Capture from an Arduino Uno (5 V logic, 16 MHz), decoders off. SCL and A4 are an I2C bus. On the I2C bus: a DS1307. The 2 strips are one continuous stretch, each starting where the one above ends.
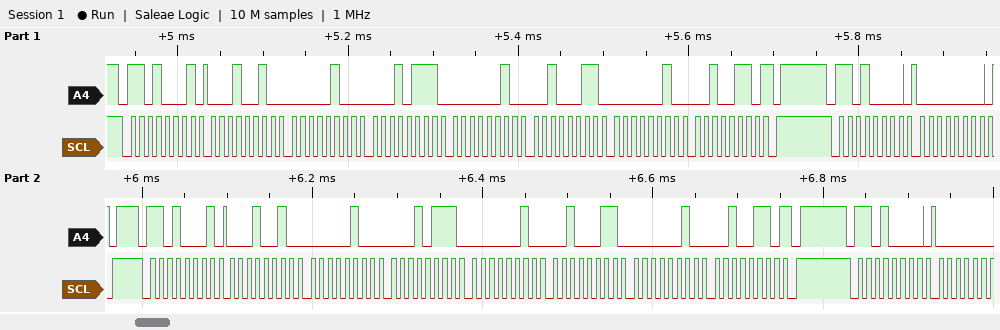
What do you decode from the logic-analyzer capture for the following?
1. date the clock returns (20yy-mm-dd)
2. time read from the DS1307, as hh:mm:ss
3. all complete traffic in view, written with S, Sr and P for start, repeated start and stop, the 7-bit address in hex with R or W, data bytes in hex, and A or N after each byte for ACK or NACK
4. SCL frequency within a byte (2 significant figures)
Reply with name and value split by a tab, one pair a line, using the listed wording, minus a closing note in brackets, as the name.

date the clock returns	2026-02-23
time read from the DS1307, as hh:mm:ss	17:04:12
all complete traffic in view, written with S, Sr and P for start, repeated start and stop, the 7-bit address in hex with R or W, data bytes in hex, and A or N after each byte for ACK or NACK	S 68R A 12 A 04 A 17 A 02 A 23 A 02 A 26 N P S 68W A 00 A P S 68R A 12 A 04 A 17 A 02 A 23 A 02 A 26 N P S 68W A
SCL frequency within a byte	100 kHz
